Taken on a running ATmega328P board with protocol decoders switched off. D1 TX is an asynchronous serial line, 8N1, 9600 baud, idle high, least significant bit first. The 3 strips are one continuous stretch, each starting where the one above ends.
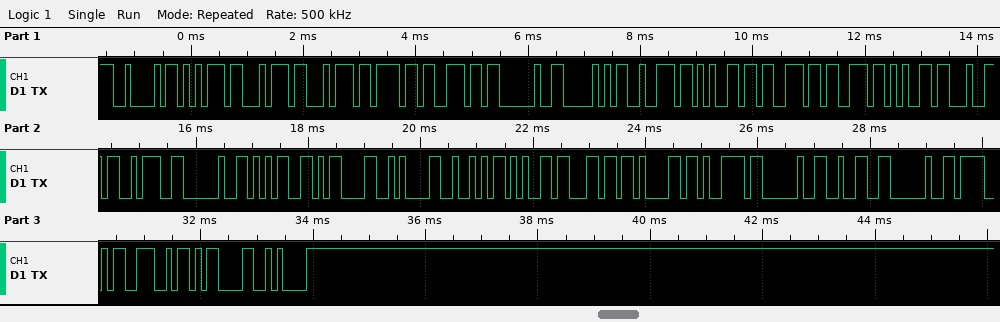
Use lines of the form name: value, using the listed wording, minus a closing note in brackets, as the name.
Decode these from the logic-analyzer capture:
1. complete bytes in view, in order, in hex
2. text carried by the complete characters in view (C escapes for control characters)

complete bytes in view, in order, in hex: 0x42 0x75 0x74 0x74 0x6F 0x6E 0x20 0x50 0x72 0x65 0x73 0x73 0x65 0x64 0x3A 0x20 0x35 0x0D 0x0A 0x52 0x65 0x6C 0x61 0x79 0x20 0x32 0x20 0x4F 0x4E 0x0D 0x0A
text carried by the complete characters in view: "Button Pressed: 5\r\nRelay 2 ON\r\n"
